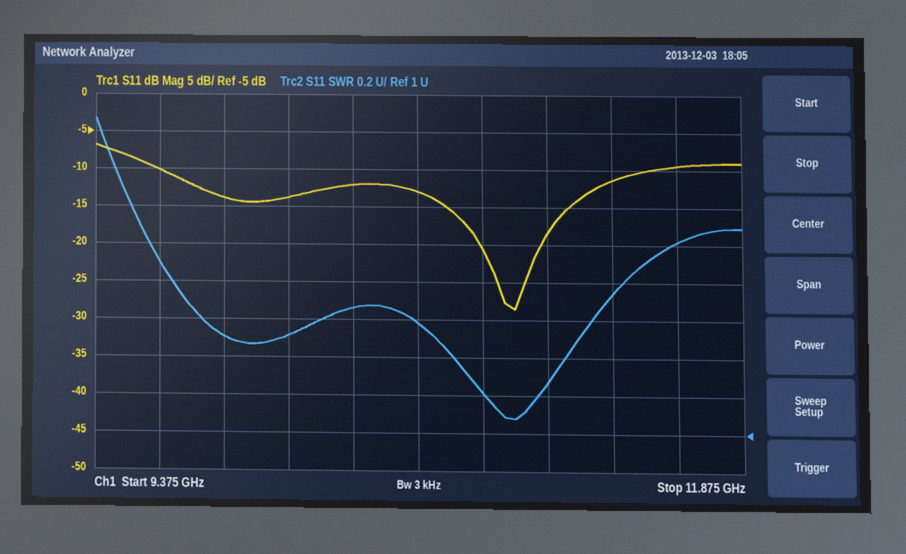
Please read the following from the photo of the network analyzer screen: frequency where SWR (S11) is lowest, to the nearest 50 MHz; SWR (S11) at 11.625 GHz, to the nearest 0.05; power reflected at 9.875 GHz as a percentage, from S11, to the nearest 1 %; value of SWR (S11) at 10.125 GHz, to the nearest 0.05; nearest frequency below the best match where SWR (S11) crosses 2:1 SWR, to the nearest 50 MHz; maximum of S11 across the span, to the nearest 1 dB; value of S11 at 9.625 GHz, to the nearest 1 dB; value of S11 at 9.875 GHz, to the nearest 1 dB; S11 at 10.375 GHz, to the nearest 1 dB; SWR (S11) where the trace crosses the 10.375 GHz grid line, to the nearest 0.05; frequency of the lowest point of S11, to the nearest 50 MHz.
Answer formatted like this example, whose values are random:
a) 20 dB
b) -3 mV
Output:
a) 11.00 GHz
b) 2.00
c) 4 %
d) 1.50
e) 9.60 GHz
f) -7 dB
g) -10 dB
h) -14 dB
i) -12 dB
j) 1.65
k) 11.00 GHz
